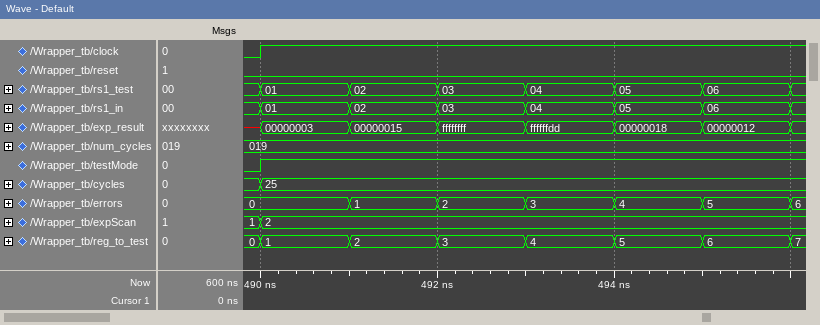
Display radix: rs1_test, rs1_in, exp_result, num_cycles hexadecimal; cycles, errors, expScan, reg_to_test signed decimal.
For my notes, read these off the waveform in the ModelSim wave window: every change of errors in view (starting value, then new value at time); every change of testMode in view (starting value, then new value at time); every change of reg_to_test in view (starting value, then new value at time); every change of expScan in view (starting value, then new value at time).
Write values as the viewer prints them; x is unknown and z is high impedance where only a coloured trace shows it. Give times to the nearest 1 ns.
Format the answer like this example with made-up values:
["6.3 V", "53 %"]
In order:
["0, 1 at 491 ns, 2 at 492 ns, 3 at 493 ns, 4 at 494 ns, 5 at 495 ns, 6 at 496 ns", "0, 1 at 490 ns", "0, 1 at 490 ns, 2 at 491 ns, 3 at 492 ns, 4 at 493 ns, 5 at 494 ns, 6 at 495 ns, 7 at 496 ns", "1, 2 at 490 ns"]
